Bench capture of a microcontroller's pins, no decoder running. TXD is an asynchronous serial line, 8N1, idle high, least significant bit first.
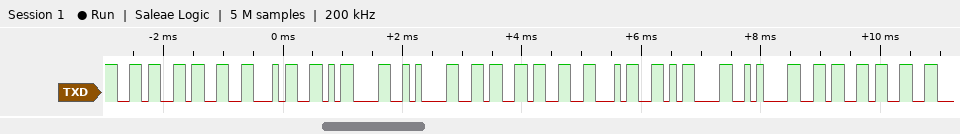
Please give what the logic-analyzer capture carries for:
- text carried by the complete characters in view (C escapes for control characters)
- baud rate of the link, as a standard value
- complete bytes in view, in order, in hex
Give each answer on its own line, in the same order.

"634\r\n634\r\n63"
9600 baud
0x36 0x33 0x34 0x0D 0x0A 0x36 0x33 0x34 0x0D 0x0A 0x36 0x33
